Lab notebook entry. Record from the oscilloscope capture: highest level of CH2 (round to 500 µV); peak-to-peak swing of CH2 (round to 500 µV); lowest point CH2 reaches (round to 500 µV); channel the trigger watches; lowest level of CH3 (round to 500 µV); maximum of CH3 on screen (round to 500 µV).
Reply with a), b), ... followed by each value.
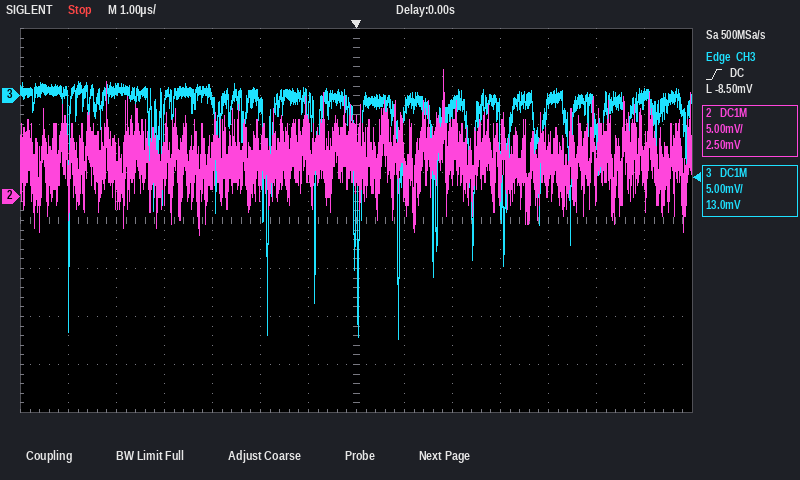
a) 13.0 mV
b) 17.0 mV
c) -4.0 mV
d) CH3
e) -25.5 mV
f) 1.5 mV
